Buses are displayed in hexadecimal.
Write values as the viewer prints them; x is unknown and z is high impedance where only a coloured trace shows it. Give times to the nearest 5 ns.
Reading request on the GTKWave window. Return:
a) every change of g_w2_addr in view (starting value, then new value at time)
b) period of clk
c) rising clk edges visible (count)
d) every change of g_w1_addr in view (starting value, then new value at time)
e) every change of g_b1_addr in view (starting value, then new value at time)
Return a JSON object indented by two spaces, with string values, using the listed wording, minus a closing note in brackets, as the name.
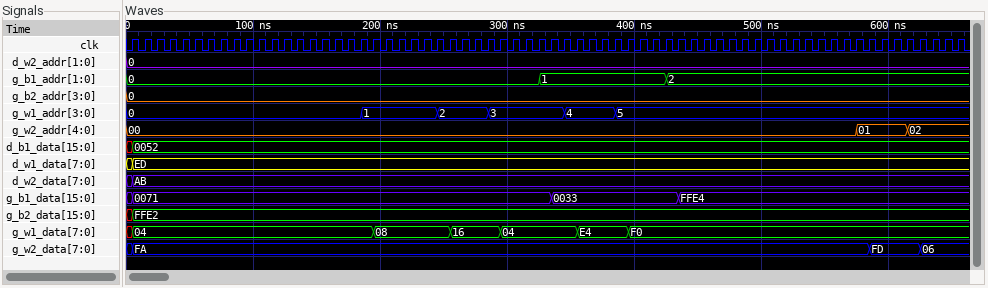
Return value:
{
  "every change of g_w2_addr in view": "00, 01 at 575 ns, 02 at 615 ns",
  "period of clk": "10 ns",
  "rising clk edges visible": "66",
  "every change of g_w1_addr in view": "0, 1 at 185 ns, 2 at 245 ns, 3 at 285 ns, 4 at 345 ns, 5 at 385 ns",
  "every change of g_b1_addr in view": "0, 1 at 325 ns, 2 at 425 ns"
}
